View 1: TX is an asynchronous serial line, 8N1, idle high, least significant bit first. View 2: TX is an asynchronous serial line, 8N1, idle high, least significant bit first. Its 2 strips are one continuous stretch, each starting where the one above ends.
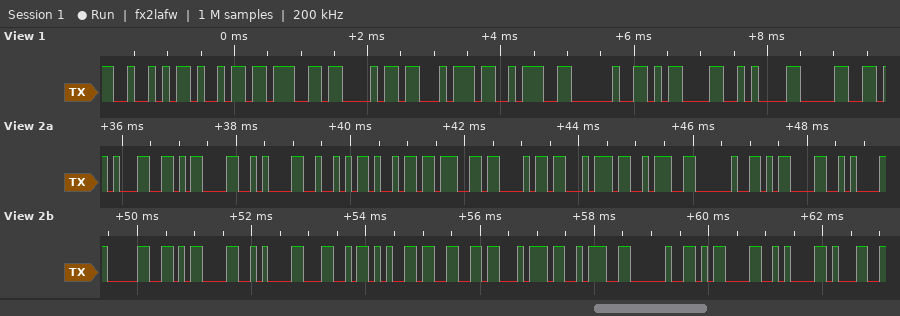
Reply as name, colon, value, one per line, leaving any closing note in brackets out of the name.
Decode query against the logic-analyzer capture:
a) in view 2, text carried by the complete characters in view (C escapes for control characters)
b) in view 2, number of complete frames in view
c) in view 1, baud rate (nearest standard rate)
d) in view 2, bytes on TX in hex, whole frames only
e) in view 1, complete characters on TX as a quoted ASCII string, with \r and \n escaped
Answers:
in view 2, text carried by the complete characters in view: "1\r\nRight: \r\n0\r\nLeft: \r\n1"
in view 2, number of complete frames in view: 24
in view 1, baud rate: 9600 baud
in view 2, bytes on TX in hex, whole frames only: 0x31 0x0D 0x0A 0x52 0x69 0x67 0x68 0x74 0x3A 0x20 0x0D 0x0A 0x30 0x0D 0x0A 0x4C 0x65 0x66 0x74 0x3A 0x20 0x0D 0x0A 0x31
in view 1, complete characters on TX as a quoted ASCII string, with \r and \n escaped: "Right: \r\n0"
